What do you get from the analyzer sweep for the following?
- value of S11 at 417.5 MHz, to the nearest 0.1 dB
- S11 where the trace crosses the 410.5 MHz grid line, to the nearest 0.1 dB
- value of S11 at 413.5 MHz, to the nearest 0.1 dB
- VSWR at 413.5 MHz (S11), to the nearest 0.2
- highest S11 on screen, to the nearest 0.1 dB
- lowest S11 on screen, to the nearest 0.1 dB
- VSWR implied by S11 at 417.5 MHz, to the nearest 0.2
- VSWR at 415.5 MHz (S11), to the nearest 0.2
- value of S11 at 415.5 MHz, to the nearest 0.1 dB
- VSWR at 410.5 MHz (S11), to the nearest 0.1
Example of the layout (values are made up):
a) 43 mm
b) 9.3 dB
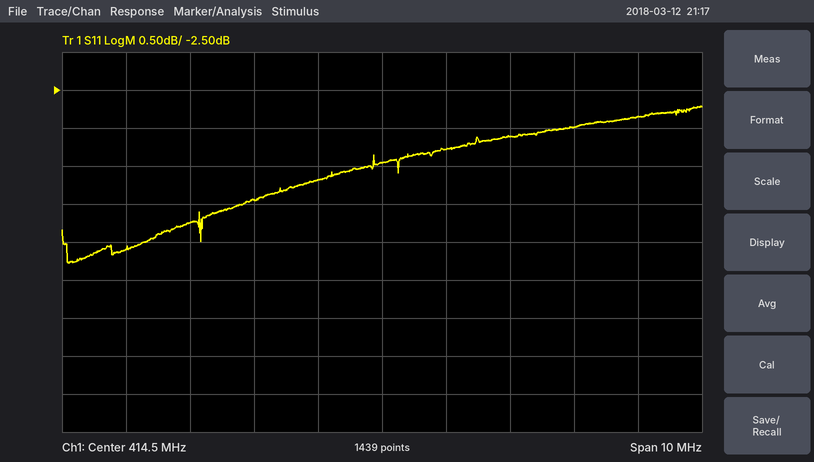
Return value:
a) -3.0 dB
b) -4.6 dB
c) -3.7 dB
d) 4.8
e) -2.7 dB
f) -4.8 dB
g) 5.8
h) 5.4
i) -3.3 dB
j) 3.9
